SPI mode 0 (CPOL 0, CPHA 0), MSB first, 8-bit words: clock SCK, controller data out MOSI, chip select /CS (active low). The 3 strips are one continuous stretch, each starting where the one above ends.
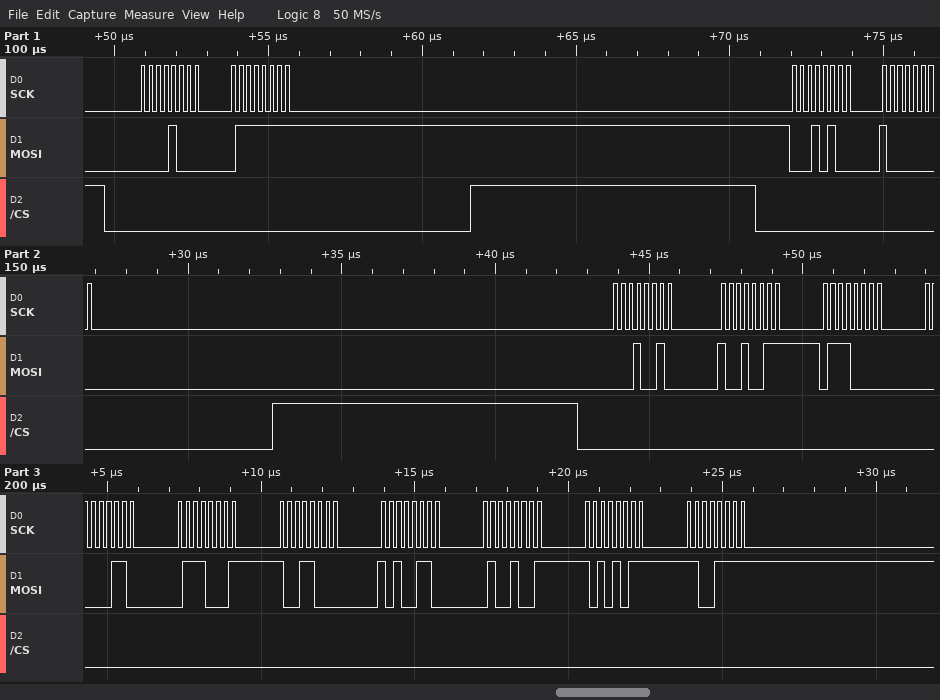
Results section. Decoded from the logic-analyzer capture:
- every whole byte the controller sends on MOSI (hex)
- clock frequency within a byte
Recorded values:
08 7F 14 80 12 93 70 06 71 98 A6 49 AB CF
4 MHz
